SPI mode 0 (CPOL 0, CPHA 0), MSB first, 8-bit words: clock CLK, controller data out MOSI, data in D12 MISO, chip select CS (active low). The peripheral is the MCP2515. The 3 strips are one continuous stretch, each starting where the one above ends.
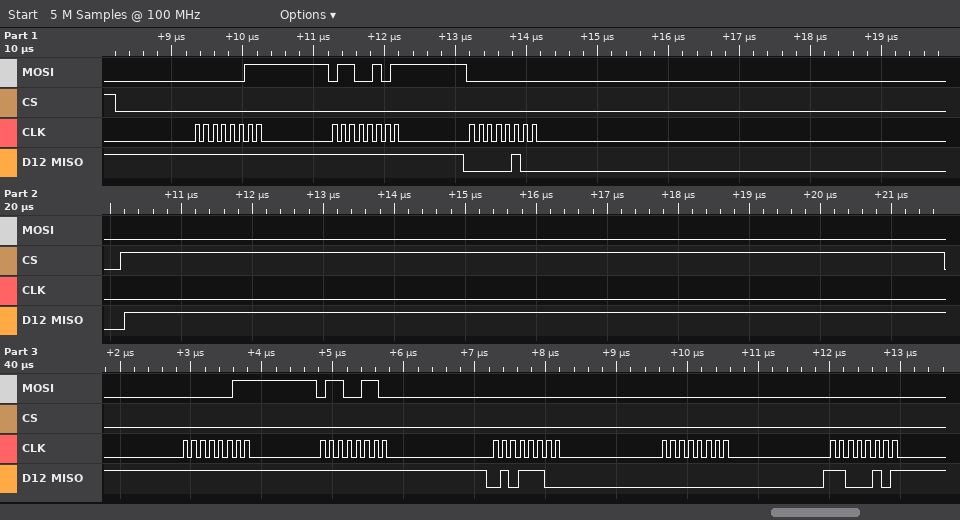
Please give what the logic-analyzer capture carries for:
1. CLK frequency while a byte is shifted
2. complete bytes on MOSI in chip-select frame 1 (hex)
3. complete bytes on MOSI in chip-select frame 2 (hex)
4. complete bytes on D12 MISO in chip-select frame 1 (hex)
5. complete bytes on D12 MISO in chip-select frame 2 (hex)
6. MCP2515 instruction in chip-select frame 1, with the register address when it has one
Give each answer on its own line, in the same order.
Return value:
8 MHz
03 65 00
03 66 00 00 00
FF FF 04
FF FF 5C 00 C5
READ 0x65
